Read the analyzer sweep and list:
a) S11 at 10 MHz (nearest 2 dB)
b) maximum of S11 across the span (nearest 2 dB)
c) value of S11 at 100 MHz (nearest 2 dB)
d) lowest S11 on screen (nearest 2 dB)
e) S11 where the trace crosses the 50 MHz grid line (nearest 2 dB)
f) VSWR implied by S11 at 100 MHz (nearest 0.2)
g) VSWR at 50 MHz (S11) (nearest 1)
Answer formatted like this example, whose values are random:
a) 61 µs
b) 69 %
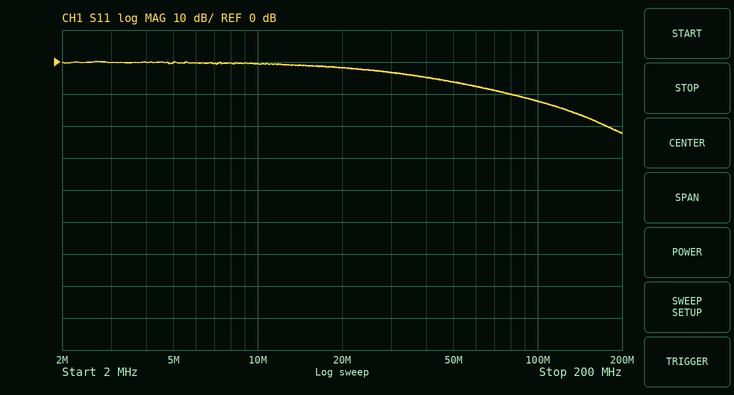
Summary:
a) 0 dB
b) 0 dB
c) -12 dB
d) -22 dB
e) -6 dB
f) 1.6
g) 3
